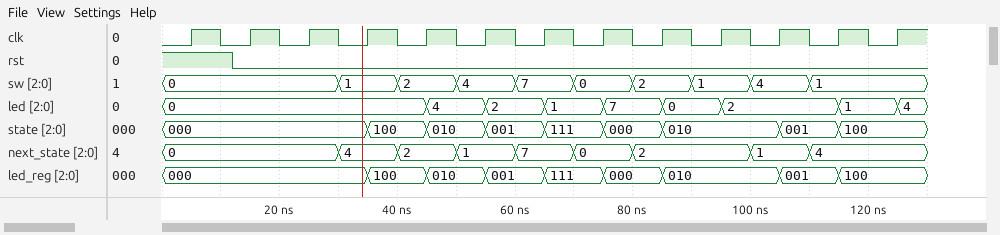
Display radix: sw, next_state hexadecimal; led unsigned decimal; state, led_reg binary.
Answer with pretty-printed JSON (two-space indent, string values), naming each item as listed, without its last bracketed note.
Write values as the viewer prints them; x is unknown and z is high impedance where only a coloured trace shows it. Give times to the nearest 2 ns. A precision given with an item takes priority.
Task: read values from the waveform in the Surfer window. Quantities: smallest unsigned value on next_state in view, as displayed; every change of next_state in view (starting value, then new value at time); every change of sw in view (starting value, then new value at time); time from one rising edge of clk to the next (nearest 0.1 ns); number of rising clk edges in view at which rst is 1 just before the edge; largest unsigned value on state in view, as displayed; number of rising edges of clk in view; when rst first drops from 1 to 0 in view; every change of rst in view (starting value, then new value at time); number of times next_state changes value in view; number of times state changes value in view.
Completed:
{
  "smallest unsigned value on next_state in view, as displayed": "0",
  "every change of next_state in view": "0, 4 at 30 ns, 2 at 40 ns, 1 at 50 ns, 7 at 60 ns, 0 at 70 ns, 2 at 80 ns, 1 at 100 ns, 4 at 110 ns",
  "every change of sw in view": "0, 1 at 30 ns, 2 at 40 ns, 4 at 50 ns, 7 at 60 ns, 0 at 70 ns, 2 at 80 ns, 1 at 90 ns, 4 at 100 ns, 1 at 110 ns",
  "time from one rising edge of clk to the next": "10 ns",
  "number of rising clk edges in view at which rst is 1 just before the edge": "1",
  "largest unsigned value on state in view, as displayed": "111",
  "number of rising edges of clk in view": "13",
  "when rst first drops from 1 to 0 in view": "12 ns",
  "every change of rst in view": "1, 0 at 12 ns",
  "number of times next_state changes value in view": "8",
  "number of times state changes value in view": "8"
}
